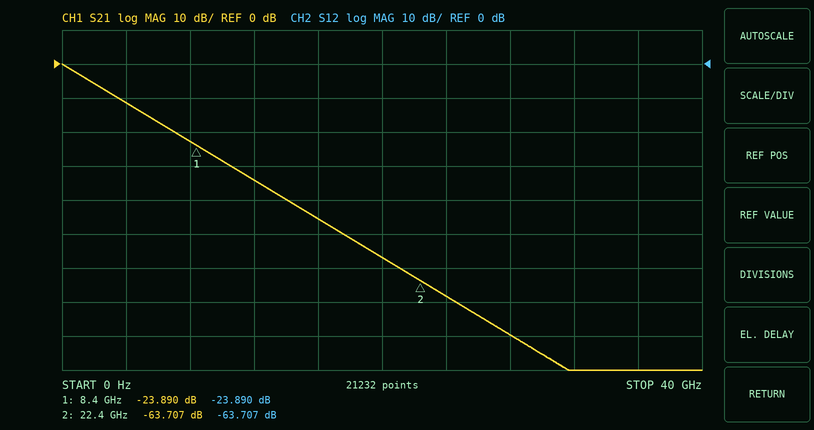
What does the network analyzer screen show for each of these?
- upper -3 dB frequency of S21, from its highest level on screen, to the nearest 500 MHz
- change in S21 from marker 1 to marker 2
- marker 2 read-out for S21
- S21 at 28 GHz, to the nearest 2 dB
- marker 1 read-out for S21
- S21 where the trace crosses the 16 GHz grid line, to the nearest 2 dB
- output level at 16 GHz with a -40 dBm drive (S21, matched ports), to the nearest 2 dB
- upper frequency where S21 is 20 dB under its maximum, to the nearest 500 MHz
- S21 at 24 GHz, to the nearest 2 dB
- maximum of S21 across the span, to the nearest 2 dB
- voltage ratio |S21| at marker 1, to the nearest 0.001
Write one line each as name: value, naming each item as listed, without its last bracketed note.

upper -3 dB frequency of S21, from its highest level on screen, to the nearest 500 MHz: 1.0 GHz
change in S21 from marker 1 to marker 2: -39.817 dB
marker 2 read-out for S21: -63.707 dB
S21 at 28 GHz, to the nearest 2 dB: -80 dB
marker 1 read-out for S21: -23.890 dB
S21 where the trace crosses the 16 GHz grid line, to the nearest 2 dB: -46 dB
output level at 16 GHz with a -40 dBm drive (S21, matched ports), to the nearest 2 dB: -86 dBm
upper frequency where S21 is 20 dB under its maximum, to the nearest 500 MHz: 7.0 GHz
S21 at 24 GHz, to the nearest 2 dB: -68 dB
maximum of S21 across the span, to the nearest 2 dB: 0 dB
voltage ratio |S21| at marker 1, to the nearest 0.001: 0.064
